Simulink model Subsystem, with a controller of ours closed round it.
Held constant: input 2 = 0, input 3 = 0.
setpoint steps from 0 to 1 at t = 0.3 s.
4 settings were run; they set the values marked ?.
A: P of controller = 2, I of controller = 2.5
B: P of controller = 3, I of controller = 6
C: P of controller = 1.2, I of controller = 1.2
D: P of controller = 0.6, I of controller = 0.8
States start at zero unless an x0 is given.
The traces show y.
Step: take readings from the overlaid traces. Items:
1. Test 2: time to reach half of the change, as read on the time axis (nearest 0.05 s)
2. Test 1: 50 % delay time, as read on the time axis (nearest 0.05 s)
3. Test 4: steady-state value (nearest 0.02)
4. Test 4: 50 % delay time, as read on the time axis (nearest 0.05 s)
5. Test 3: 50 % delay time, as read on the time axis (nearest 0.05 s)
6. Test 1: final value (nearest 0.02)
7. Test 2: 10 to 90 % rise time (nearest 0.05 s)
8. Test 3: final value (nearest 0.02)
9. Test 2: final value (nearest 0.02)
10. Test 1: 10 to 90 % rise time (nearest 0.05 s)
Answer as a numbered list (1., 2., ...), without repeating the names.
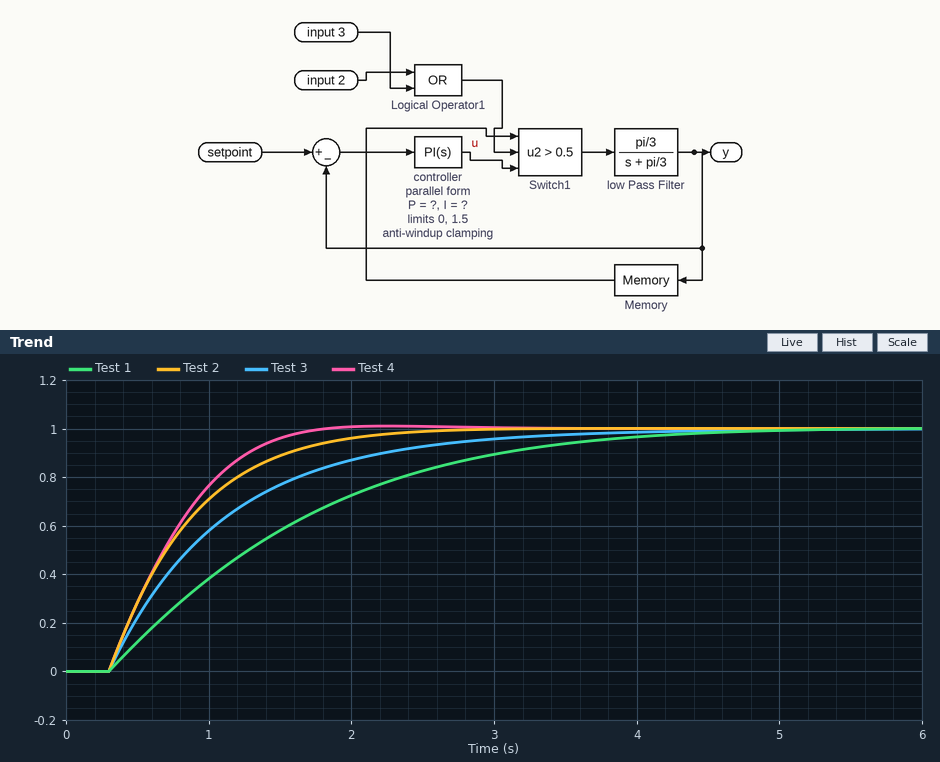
1. 0.70 s
2. 1.30 s
3. 1.00
4. 0.70 s
5. 0.85 s
6. 1.00
7. 1.20 s
8. 1.00
9. 1.00
10. 2.60 s
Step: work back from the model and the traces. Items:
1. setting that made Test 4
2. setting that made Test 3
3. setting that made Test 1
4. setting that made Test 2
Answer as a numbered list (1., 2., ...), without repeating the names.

1. B
2. C
3. D
4. A
